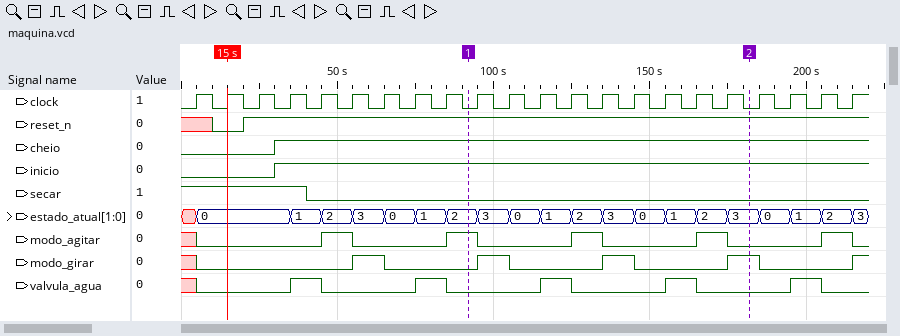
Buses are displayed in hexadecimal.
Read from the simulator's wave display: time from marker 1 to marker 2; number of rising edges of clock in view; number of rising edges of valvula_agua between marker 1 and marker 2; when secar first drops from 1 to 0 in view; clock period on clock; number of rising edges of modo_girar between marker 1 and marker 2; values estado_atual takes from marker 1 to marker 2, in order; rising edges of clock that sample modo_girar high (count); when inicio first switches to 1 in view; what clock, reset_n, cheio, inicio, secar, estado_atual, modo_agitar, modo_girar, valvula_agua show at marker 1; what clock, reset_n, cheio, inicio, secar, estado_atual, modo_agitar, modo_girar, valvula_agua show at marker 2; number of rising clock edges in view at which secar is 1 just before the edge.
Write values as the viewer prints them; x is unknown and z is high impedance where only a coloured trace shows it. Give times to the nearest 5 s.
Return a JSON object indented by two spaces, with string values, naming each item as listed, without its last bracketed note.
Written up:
{
  "time from marker 1 to marker 2": "90 s",
  "number of rising edges of clock in view": "22",
  "number of rising edges of valvula_agua between marker 1 and marker 2": "2",
  "when secar first drops from 1 to 0 in view": "40 s",
  "clock period on clock": "10 s",
  "number of rising edges of modo_girar between marker 1 and marker 2": "3",
  "values estado_atual takes from marker 1 to marker 2, in order": "2, 3, 0, 1, 2, 3, 0, 1, 2, 3",
  "rising edges of clock that sample modo_girar high": "4",
  "when inicio first switches to 1 in view": "30 s",
  "what clock, reset_n, cheio, inicio, secar, estado_atual, modo_agitar, modo_girar, valvula_agua show at marker 1": "clock=0, reset_n=1, cheio=1, inicio=1, secar=0, estado_atual=2, modo_agitar=1, modo_girar=0, valvula_agua=0",
  "what clock, reset_n, cheio, inicio, secar, estado_atual, modo_agitar, modo_girar, valvula_agua show at marker 2": "clock=0, reset_n=1, cheio=1, inicio=1, secar=0, estado_atual=3, modo_agitar=0, modo_girar=1, valvula_agua=0",
  "number of rising clock edges in view at which secar is 1 just before the edge": "4"
}
